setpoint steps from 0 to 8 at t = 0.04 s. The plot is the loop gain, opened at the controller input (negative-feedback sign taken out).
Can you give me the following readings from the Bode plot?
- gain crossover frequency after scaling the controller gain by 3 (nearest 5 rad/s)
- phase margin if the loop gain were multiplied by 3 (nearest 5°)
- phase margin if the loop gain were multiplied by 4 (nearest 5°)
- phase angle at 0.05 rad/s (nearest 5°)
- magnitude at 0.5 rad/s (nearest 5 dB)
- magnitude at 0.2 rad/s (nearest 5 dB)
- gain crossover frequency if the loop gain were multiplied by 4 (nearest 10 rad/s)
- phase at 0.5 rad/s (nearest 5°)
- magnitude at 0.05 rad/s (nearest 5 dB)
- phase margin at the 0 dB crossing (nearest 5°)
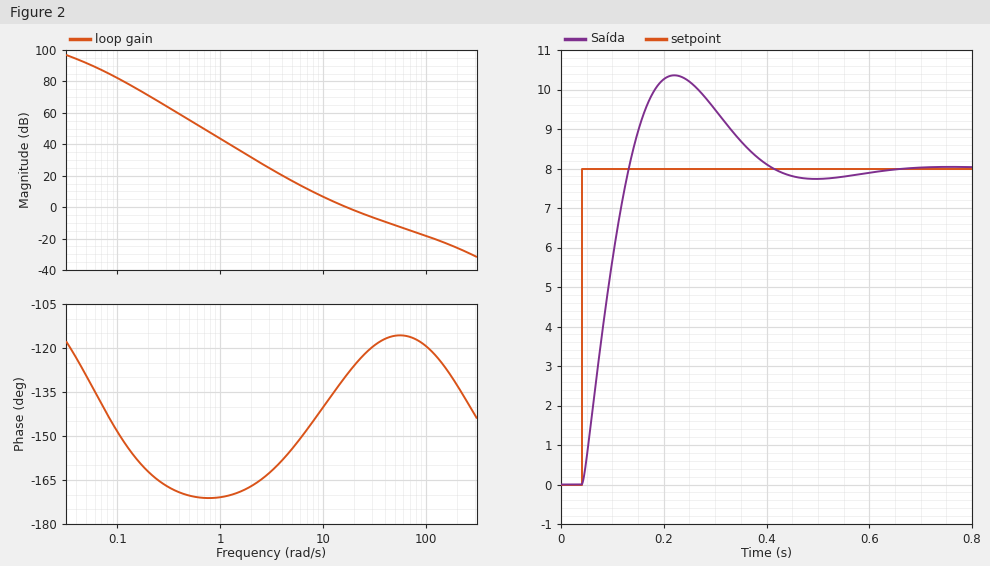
40 rad/s
65°
65°
-130°
55 dB
70 dB
50 rad/s
-170°
90 dB
50°
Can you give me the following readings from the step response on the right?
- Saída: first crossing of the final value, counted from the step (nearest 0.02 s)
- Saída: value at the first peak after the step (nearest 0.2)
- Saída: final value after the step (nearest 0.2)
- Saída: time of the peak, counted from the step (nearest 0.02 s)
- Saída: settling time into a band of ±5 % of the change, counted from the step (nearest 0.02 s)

0.10 s
10.4
8.0
0.18 s
0.34 s
